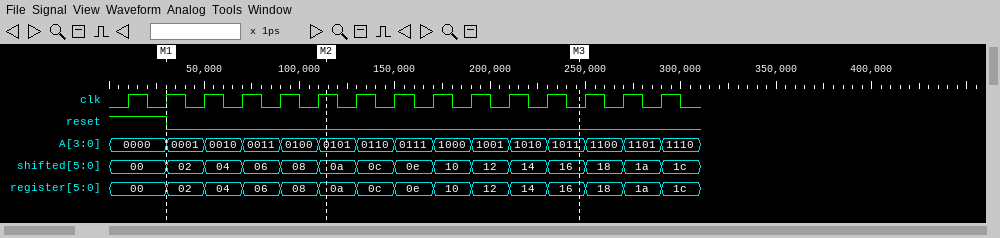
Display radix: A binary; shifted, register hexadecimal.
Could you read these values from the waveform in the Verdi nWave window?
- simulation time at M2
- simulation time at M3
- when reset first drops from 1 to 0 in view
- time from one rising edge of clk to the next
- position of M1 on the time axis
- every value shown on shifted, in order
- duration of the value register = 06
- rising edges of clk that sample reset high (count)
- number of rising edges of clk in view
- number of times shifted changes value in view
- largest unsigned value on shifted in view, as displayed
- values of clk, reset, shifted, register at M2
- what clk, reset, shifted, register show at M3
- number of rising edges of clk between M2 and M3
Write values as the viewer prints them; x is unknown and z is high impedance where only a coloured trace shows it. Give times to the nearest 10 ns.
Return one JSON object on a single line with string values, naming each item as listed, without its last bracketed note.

{"simulation time at M2": "110 ns", "simulation time at M3": "250 ns", "when reset first drops from 1 to 0 in view": "30 ns", "time from one rising edge of clk to the next": "20 ns", "position of M1 on the time axis": "30 ns", "every value shown on shifted, in order": "00, 02, 04, 06, 08, 0a, 0c, 0e, 10, 12, 14, 16, 18, 1a, 1c", "duration of the value register = 06": "20 ns", "rising edges of clk that sample reset high": "2", "number of rising edges of clk in view": "15", "number of times shifted changes value in view": "14", "largest unsigned value on shifted in view, as displayed": "1c", "values of clk, reset, shifted, register at M2": "clk=1, reset=0, shifted=0a, register=0a", "what clk, reset, shifted, register show at M3": "clk=0, reset=0, shifted=16, register=16", "number of rising edges of clk between M2 and M3": "6"}
